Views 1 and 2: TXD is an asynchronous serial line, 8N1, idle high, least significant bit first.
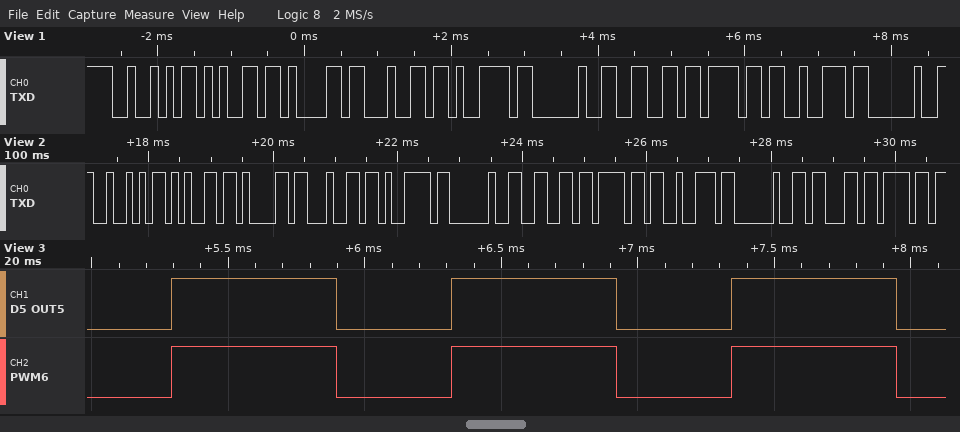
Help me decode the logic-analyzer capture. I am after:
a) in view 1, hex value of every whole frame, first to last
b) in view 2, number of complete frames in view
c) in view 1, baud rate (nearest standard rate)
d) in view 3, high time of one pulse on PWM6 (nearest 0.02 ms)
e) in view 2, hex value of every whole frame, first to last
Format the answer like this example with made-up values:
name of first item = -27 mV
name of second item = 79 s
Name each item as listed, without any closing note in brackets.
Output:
in view 1, hex value of every whole frame, first to last = 52 65 61 64 79 20 66 6F 72 20
in view 2, number of complete frames in view = 12
in view 1, baud rate = 9600 baud
in view 3, high time of one pulse on PWM6 = 0.60 ms
in view 2, hex value of every whole frame, first to last = 52 65 61 64 79 20 66 6F 72 20 63 6F
